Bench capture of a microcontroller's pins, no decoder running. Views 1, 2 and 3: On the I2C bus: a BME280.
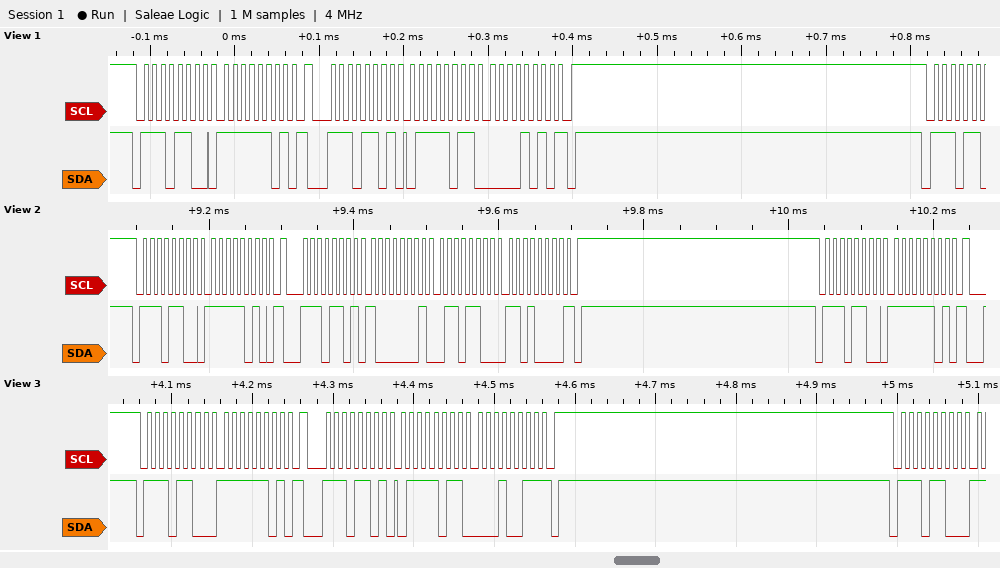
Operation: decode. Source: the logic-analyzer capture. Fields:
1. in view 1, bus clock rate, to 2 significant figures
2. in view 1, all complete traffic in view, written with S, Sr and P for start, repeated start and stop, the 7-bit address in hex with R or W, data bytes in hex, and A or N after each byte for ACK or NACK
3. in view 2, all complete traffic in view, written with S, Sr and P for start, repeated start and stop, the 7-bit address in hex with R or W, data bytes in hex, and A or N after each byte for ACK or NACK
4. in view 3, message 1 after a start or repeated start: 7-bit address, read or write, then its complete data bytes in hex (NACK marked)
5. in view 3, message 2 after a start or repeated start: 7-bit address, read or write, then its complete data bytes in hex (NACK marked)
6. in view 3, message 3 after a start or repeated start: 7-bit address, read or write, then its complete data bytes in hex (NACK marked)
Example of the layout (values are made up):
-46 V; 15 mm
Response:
100 kHz; S 76W A FD A Sr 76R A 7B A 0A N P; S 76W A FA A Sr 76R A 81 A 6C A D0 N P S 76W A FD A; 0x76 write: FD; 0x76 read: 7B 13 NACK; 0x76 write
